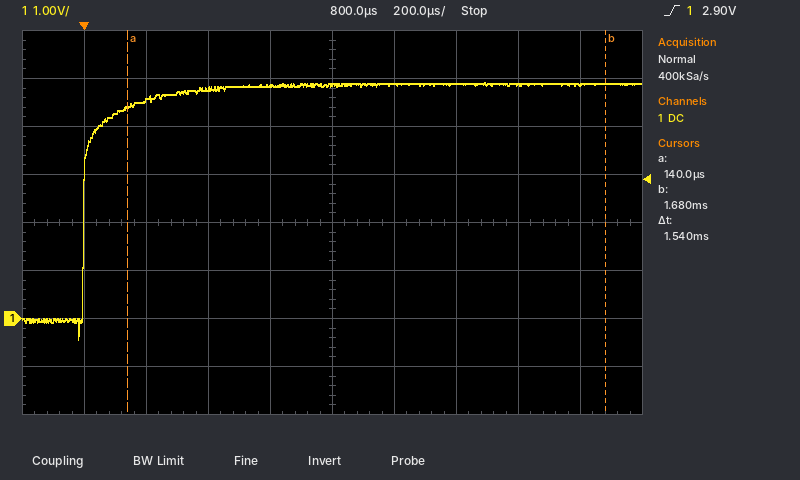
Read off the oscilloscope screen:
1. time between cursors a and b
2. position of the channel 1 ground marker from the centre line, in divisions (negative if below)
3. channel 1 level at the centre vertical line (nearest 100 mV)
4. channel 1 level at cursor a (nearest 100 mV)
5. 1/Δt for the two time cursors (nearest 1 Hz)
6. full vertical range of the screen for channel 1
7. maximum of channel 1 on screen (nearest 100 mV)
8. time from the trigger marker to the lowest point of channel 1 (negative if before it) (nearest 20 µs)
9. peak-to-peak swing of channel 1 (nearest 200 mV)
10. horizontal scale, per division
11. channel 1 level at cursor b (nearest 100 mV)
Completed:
1.54 ms
-2.0 div
4.9 V
4.4 V
649 Hz
8 V
4.9 V
-20 µs
5.4 V
200 µs
4.9 V
